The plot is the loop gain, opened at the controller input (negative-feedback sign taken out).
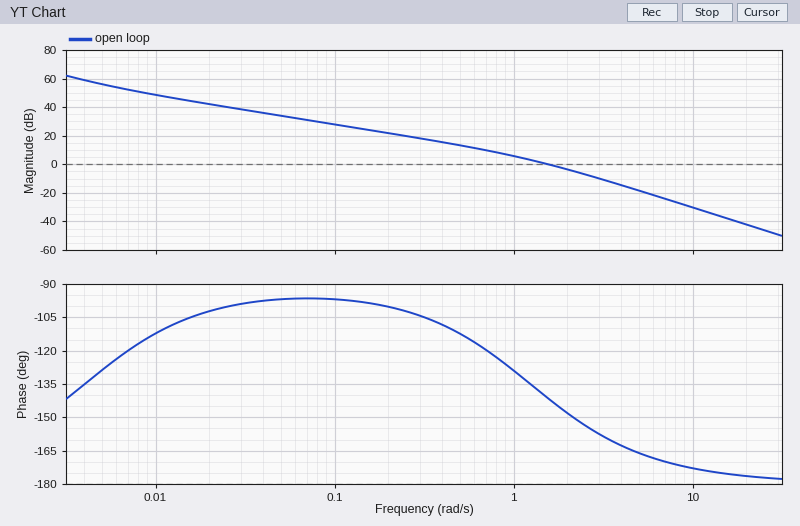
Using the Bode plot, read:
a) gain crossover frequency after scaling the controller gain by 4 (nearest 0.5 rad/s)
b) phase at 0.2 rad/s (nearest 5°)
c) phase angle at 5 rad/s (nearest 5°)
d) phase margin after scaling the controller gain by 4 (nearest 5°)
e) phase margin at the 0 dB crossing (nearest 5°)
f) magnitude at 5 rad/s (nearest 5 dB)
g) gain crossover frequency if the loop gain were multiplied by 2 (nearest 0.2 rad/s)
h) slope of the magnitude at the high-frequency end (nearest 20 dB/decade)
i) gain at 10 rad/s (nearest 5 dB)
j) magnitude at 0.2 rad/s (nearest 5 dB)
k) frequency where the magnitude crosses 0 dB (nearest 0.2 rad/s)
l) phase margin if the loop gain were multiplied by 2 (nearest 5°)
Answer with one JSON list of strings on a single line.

["3.5 rad/s", "-100°", "-165°", "20°", "40°", "-20 dB", "2.4 rad/s", "-40 dB/decade", "-30 dB", "20 dB", "1.6 rad/s", "30°"]
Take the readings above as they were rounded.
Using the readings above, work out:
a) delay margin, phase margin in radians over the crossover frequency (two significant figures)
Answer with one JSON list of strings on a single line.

["0.44 s"]
